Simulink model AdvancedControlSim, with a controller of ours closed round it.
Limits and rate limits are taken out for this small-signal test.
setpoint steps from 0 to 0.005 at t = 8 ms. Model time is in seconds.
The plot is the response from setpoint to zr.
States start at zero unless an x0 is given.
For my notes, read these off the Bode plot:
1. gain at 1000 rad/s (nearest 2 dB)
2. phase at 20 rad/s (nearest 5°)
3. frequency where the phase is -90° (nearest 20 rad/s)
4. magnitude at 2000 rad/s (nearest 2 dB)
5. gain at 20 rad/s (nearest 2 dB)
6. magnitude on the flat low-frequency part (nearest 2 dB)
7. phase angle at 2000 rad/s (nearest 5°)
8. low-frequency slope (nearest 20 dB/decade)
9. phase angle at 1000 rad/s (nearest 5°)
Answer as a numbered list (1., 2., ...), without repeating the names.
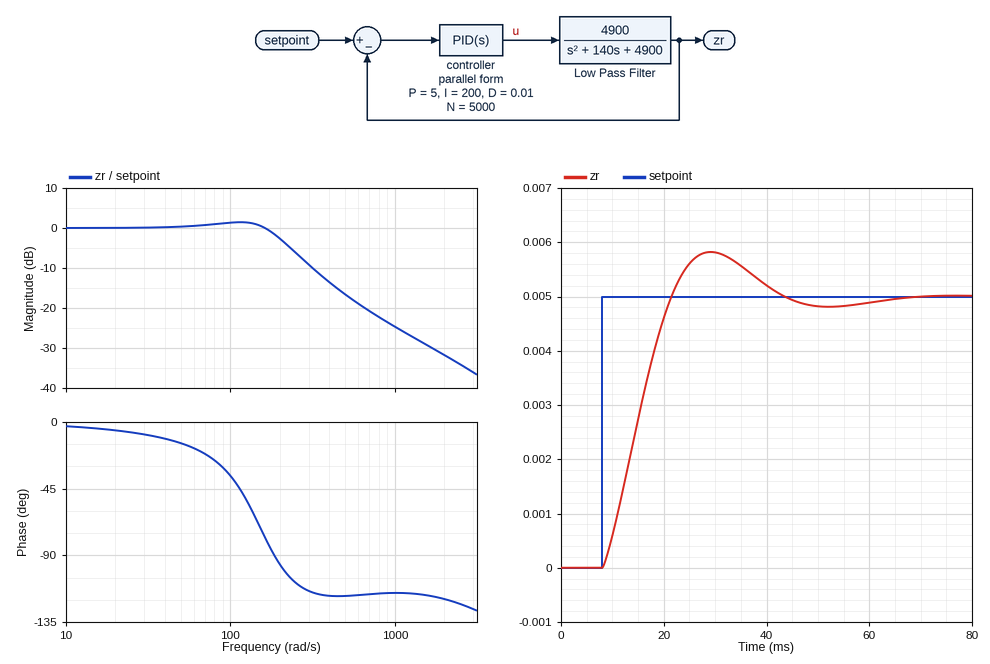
1. -24 dB
2. -5°
3. 180 rad/s
4. -32 dB
5. 0 dB
6. 0 dB
7. -120°
8. 0 dB/decade
9. -115°
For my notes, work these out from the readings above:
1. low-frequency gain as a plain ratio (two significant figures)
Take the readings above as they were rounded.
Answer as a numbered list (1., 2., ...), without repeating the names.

1. 1.0
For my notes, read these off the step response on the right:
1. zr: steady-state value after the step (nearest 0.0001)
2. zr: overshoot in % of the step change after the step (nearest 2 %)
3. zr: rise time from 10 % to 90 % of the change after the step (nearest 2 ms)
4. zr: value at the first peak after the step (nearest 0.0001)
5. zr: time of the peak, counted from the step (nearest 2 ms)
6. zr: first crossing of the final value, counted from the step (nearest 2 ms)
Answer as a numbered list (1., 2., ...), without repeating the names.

1. 0.0050
2. 16 %
3. 10 ms
4. 0.0058
5. 22 ms
6. 14 ms
